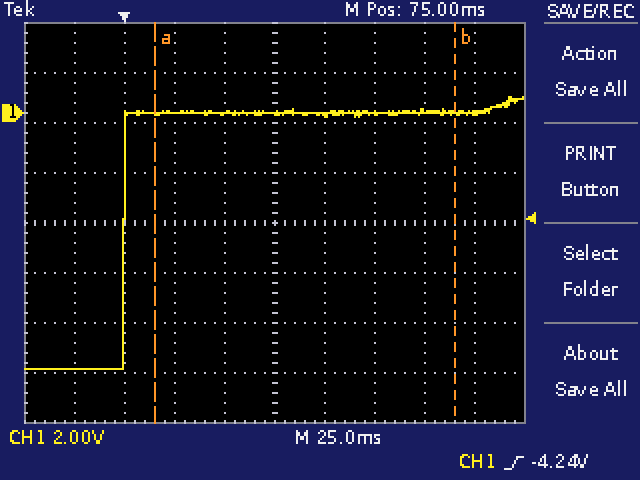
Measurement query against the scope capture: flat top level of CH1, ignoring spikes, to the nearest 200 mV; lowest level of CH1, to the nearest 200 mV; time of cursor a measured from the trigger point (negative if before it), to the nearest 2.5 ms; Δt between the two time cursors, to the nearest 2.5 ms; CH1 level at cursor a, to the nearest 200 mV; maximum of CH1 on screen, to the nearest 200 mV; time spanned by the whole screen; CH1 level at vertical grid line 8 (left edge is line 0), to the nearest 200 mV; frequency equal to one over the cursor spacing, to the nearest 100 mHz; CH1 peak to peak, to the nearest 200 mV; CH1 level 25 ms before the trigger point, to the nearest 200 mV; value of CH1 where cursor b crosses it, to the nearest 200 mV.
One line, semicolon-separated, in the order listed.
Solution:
0.0 V; -10.2 V; +15.0 ms; 150.0 ms; 0.0 V; 600 mV; 250 ms; 0.0 V; 6.7 Hz; 10.8 V; -10.2 V; 0.0 V
